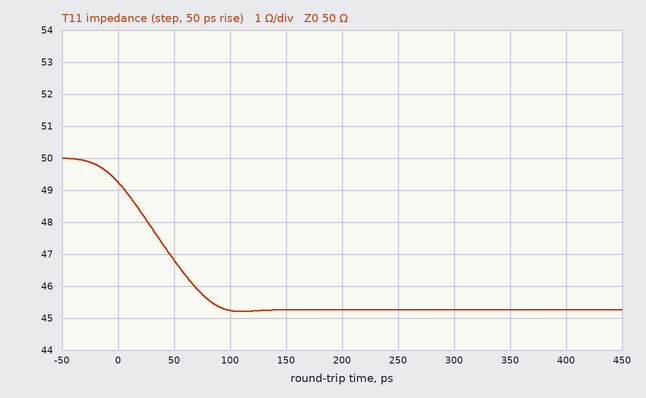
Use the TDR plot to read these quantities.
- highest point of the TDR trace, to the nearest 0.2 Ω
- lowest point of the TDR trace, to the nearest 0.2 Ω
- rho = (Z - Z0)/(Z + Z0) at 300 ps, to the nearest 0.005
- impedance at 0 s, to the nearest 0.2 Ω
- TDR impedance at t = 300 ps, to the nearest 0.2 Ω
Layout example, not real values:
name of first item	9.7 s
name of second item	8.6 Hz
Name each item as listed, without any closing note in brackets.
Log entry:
highest point of the TDR trace, to the nearest 0.2 Ω	50.0 Ω
lowest point of the TDR trace, to the nearest 0.2 Ω	45.2 Ω
rho = (Z - Z0)/(Z + Z0) at 300 ps, to the nearest 0.005	-0.050
impedance at 0 s, to the nearest 0.2 Ω	49.2 Ω
TDR impedance at t = 300 ps, to the nearest 0.2 Ω	45.2 Ω
